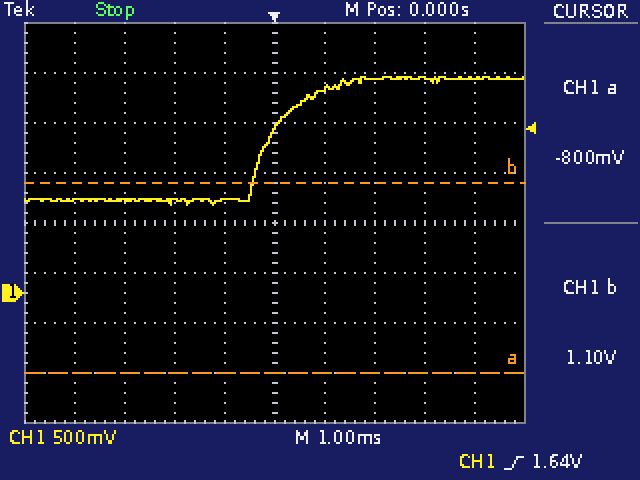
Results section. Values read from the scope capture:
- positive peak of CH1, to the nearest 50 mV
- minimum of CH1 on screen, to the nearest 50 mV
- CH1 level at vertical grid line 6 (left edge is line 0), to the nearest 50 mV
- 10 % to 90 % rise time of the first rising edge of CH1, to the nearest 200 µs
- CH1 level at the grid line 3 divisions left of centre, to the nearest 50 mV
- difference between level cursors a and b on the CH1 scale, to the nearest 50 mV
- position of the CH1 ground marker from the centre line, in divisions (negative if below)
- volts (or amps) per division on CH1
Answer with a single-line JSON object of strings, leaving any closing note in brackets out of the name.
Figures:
{"positive peak of CH1, to the nearest 50 mV": "2.15 V", "minimum of CH1 on screen, to the nearest 50 mV": "900 mV", "CH1 level at vertical grid line 6 (left edge is line 0), to the nearest 50 mV": "2.05 V", "10 % to 90 % rise time of the first rising edge of CH1, to the nearest 200 µs": "1.4 ms", "CH1 level at the grid line 3 divisions left of centre, to the nearest 50 mV": "950 mV", "difference between level cursors a and b on the CH1 scale, to the nearest 50 mV": "1.90 V", "position of the CH1 ground marker from the centre line, in divisions": "-1.4 div", "volts (or amps) per division on CH1": "500 mV"}
